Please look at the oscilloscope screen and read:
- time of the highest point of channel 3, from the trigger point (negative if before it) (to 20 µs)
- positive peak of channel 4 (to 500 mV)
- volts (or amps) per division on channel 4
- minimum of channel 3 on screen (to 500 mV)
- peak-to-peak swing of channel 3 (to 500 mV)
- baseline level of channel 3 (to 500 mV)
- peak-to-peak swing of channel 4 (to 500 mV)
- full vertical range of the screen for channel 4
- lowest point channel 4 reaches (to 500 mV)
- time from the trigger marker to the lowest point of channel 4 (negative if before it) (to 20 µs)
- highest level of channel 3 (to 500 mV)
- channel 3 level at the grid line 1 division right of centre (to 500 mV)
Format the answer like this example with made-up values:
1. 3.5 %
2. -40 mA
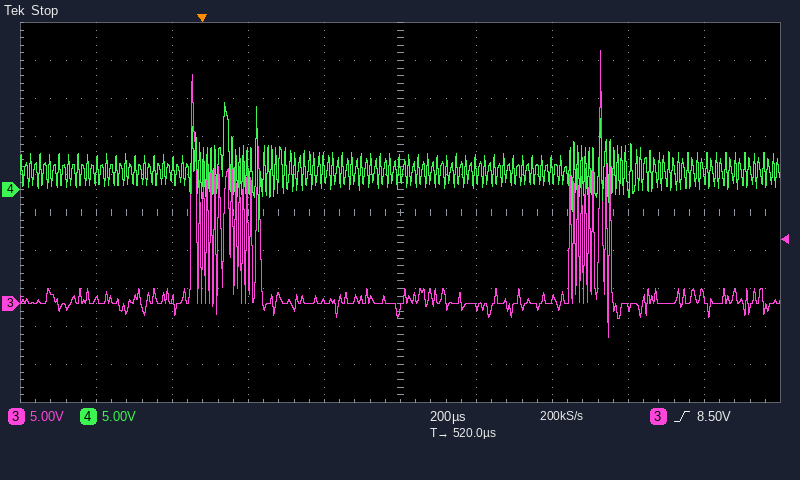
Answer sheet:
1. +1.04 ms
2. 11.5 V
3. 5 V
4. -4.5 V
5. 38.0 V
6. 0.0 V
7. 17.0 V
8. 50 V
9. -5.5 V
10. +140 µs
11. 33.5 V
12. -500 mV
